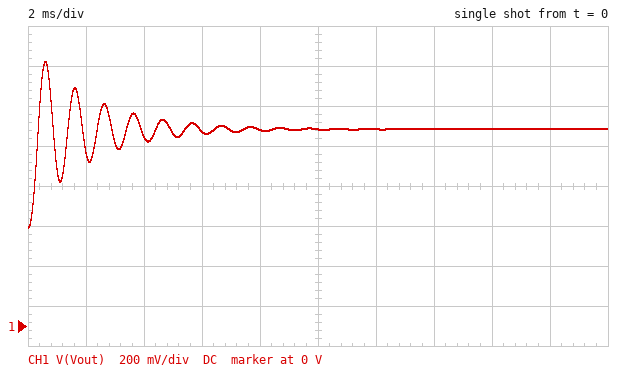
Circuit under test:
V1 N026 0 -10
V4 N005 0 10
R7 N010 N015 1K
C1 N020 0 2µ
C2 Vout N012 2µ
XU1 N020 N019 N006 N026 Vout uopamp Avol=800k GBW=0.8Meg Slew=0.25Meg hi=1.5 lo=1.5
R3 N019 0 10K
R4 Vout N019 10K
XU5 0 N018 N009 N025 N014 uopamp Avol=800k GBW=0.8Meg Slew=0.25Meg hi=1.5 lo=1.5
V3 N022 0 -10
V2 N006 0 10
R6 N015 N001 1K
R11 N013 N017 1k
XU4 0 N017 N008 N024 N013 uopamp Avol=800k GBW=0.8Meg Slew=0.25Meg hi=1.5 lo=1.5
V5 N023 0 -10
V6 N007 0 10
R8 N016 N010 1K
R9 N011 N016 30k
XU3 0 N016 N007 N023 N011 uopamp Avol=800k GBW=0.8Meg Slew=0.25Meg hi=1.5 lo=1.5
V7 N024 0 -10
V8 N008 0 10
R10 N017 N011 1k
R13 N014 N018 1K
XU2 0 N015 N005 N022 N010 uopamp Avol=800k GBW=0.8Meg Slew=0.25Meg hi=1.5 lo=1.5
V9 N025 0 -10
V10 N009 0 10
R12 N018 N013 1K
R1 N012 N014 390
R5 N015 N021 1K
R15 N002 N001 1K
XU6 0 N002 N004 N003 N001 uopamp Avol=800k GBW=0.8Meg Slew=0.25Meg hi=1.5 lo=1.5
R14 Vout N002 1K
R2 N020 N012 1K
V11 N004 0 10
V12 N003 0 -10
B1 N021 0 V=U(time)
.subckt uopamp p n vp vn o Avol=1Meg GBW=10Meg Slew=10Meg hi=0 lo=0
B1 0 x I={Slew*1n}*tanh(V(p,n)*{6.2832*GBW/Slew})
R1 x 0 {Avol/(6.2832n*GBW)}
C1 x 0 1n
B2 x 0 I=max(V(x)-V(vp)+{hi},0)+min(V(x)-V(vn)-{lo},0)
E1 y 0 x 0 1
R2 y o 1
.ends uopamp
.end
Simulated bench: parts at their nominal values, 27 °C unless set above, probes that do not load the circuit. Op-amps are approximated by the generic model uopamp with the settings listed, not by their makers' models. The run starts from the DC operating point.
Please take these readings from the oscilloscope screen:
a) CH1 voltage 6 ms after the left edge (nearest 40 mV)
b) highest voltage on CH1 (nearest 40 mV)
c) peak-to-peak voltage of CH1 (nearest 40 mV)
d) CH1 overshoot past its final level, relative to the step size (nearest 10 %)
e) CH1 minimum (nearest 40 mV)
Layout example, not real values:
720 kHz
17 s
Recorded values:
960 mV
1.32 V
840 mV
70 %
480 mV
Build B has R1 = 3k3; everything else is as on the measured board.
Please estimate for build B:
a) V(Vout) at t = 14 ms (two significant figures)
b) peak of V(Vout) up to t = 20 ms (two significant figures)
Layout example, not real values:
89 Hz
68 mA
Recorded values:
1.2 V
1.4 V
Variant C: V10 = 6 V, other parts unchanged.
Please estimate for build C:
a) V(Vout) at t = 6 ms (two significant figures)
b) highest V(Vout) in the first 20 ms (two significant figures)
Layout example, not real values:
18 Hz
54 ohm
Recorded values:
1.0 V
1.2 V
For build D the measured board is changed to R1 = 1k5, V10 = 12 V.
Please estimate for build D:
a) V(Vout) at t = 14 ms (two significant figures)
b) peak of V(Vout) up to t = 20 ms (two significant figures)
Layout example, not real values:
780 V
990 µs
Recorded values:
910 mV
1.4 V
